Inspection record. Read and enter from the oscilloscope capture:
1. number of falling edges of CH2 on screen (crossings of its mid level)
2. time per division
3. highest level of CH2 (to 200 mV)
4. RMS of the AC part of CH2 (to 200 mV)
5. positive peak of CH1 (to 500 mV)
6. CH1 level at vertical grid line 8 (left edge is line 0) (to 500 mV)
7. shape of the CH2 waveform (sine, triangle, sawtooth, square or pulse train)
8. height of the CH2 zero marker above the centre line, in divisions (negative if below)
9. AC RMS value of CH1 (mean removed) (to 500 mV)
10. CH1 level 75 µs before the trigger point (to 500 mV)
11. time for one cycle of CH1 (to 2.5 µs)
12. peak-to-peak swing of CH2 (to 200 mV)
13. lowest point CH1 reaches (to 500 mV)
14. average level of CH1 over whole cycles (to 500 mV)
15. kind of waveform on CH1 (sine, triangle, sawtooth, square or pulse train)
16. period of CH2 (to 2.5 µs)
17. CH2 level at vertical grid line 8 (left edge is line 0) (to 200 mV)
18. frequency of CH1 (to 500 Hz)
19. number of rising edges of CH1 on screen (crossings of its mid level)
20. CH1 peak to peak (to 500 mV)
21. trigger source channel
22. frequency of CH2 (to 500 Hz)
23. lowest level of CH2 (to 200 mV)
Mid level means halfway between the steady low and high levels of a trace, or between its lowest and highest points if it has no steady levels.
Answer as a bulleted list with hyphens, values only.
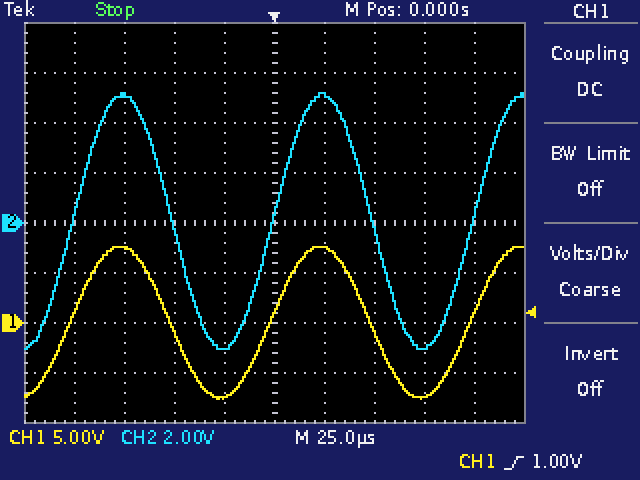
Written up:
- 2
- 25 µs
- 5.2 V
- 3.6 V
- 7.5 V
- -7.5 V
- sine
- 0.0 div
- 5.5 V
- 7.5 V
- 100.0 µs
- 10.2 V
- -7.5 V
- 0.0 V
- sine
- 100.0 µs
- -5.0 V
- 10.0 kHz
- 3
- 15.0 V
- CH1
- 10.0 kHz
- -5.0 V
